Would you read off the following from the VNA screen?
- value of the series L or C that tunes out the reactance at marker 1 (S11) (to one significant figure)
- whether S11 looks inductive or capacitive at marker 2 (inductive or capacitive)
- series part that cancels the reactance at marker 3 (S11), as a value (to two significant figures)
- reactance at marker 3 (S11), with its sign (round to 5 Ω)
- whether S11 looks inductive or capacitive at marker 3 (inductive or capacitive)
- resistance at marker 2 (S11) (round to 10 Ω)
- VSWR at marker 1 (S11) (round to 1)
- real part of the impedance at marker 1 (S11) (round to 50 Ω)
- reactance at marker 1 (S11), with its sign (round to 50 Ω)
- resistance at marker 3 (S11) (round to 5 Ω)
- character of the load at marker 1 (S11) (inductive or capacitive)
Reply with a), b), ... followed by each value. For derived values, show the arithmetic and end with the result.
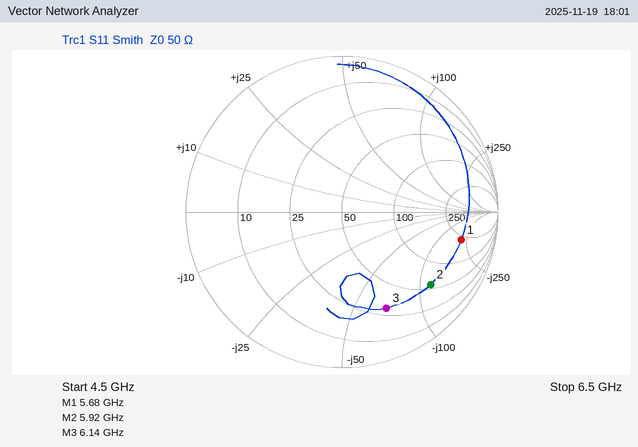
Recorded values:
a) L = 200 Ω/(2π × 5.68 GHz) ≈ 6 nH
b) capacitive
c) L = 70 Ω/(2π × 6.14 GHz) ≈ 1.8 nH
d) -70 Ω
e) capacitive
f) 60 Ω
g) 8
h) 200 Ω
i) -200 Ω
j) 30 Ω
k) capacitive
